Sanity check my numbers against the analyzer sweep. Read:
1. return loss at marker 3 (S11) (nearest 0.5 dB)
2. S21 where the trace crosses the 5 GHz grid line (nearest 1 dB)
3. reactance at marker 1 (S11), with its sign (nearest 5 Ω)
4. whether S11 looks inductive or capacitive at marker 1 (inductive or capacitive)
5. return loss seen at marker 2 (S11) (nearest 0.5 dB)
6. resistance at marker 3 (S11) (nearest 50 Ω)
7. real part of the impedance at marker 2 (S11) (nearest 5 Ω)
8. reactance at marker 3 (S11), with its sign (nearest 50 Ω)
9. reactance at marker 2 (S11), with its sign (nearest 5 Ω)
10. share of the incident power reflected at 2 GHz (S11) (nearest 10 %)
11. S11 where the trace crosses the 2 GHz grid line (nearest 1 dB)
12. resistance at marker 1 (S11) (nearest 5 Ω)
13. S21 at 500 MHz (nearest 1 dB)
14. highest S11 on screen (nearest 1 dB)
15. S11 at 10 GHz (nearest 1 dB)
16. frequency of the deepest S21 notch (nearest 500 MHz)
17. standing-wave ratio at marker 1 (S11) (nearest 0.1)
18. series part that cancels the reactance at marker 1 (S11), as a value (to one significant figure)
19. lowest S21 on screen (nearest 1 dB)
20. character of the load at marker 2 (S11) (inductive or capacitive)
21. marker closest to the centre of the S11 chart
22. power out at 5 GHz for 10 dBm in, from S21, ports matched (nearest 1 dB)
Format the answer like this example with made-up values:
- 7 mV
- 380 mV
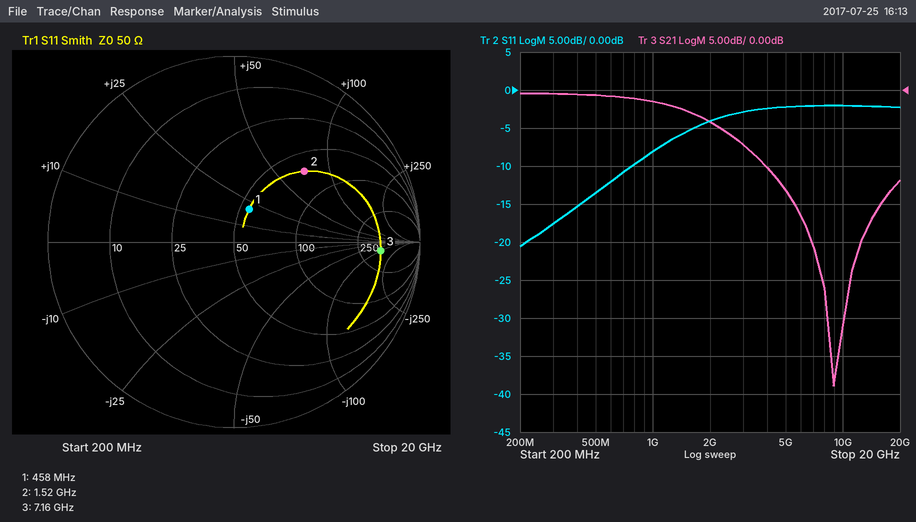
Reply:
- 2.0 dB
- -13 dB
- +20 Ω
- inductive
- 5.5 dB
- 400 Ω
- 65 Ω
- -100 Ω
- +70 Ω
- 40 %
- -4 dB
- 55 Ω
- -1 dB
- -2 dB
- -2 dB
- 9.0 GHz
- 1.5
- 20 pF
- -39 dB
- inductive
- marker 1
- -3 dBm
